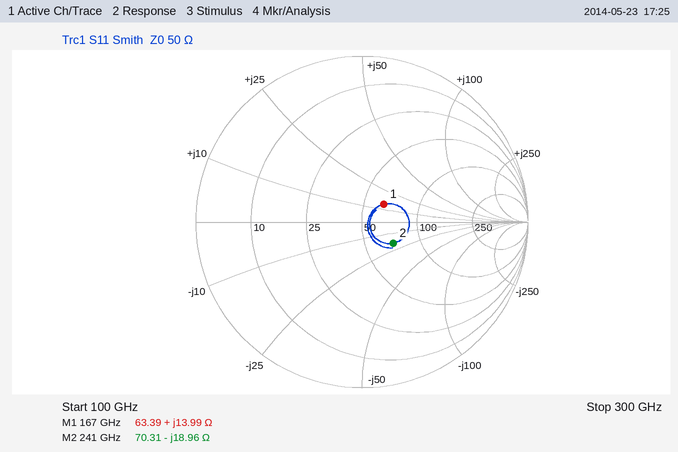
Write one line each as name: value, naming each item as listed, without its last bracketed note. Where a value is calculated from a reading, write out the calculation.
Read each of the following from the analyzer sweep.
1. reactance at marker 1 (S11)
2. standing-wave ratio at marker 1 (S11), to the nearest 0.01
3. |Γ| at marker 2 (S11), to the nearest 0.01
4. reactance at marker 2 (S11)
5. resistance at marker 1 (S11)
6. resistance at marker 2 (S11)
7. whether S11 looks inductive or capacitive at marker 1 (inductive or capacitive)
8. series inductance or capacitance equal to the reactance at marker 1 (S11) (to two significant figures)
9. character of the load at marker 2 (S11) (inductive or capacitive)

reactance at marker 1: +13.99 Ω
standing-wave ratio at marker 1 (S11), to the nearest 0.01: 1.41
|Γ| at marker 2 (S11), to the nearest 0.01: 0.23
reactance at marker 2: -18.96 Ω
resistance at marker 1: 63.39 Ω
resistance at marker 2: 70.31 Ω
whether S11 looks inductive or capacitive at marker 1: inductive
series inductance or capacitance equal to the reactance at marker 1 (S11): L = 13.99 Ω/(2π × 167 GHz) ≈ 13 pH
character of the load at marker 2 (S11): capacitive
